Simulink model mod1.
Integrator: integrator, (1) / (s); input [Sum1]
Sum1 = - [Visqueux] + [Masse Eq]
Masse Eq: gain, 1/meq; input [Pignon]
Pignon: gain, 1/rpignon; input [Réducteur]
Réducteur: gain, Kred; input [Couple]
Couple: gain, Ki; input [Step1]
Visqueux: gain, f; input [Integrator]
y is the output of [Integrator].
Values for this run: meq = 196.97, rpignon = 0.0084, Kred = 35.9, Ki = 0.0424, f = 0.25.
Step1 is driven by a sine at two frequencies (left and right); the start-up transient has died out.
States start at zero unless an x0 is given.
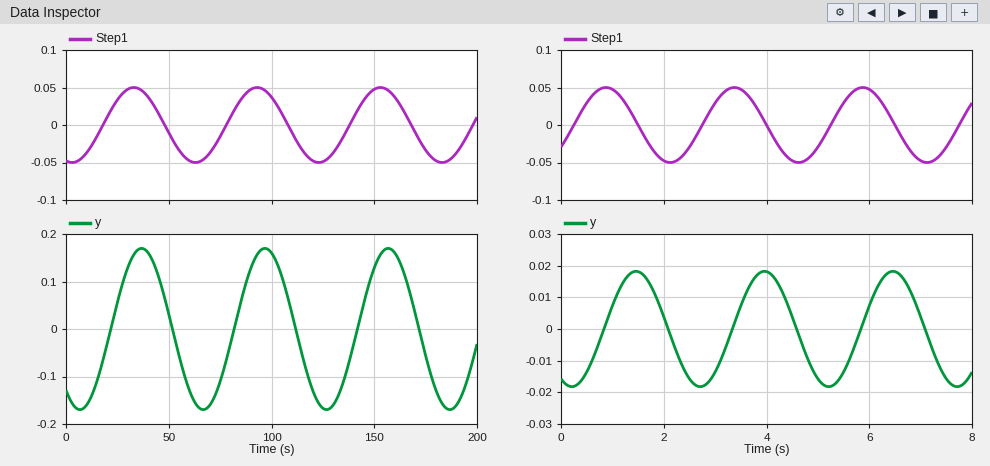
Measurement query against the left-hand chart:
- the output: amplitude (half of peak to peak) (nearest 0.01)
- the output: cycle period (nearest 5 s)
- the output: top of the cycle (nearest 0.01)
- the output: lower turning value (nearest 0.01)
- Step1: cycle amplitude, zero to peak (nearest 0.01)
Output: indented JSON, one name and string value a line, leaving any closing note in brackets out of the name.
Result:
{
  "the output: amplitude (half of peak to peak)": "0.17",
  "the output: cycle period": "60 s",
  "the output: top of the cycle": "0.17",
  "the output: lower turning value": "-0.17",
  "Step1: cycle amplitude, zero to peak": "0.05"
}
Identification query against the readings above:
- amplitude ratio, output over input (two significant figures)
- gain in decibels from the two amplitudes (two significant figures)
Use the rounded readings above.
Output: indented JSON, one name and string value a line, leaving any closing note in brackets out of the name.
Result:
{
  "amplitude ratio, output over input": "3.4",
  "gain in decibels from the two amplitudes": "11 dB"
}
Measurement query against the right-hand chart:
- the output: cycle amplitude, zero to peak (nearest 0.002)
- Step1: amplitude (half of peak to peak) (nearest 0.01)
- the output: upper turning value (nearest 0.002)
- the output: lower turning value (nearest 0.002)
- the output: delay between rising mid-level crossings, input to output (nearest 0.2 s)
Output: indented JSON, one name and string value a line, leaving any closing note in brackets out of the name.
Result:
{
  "the output: cycle amplitude, zero to peak": "0.018",
  "Step1: amplitude (half of peak to peak)": "0.05",
  "the output: upper turning value": "0.018",
  "the output: lower turning value": "-0.018",
  "the output: delay between rising mid-level crossings, input to output": "0.6 s"
}
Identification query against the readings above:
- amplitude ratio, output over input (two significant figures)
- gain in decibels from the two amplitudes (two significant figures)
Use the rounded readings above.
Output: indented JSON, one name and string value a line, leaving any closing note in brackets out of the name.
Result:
{
  "amplitude ratio, output over input": "0.36",
  "gain in decibels from the two amplitudes": "-8.9 dB"
}
